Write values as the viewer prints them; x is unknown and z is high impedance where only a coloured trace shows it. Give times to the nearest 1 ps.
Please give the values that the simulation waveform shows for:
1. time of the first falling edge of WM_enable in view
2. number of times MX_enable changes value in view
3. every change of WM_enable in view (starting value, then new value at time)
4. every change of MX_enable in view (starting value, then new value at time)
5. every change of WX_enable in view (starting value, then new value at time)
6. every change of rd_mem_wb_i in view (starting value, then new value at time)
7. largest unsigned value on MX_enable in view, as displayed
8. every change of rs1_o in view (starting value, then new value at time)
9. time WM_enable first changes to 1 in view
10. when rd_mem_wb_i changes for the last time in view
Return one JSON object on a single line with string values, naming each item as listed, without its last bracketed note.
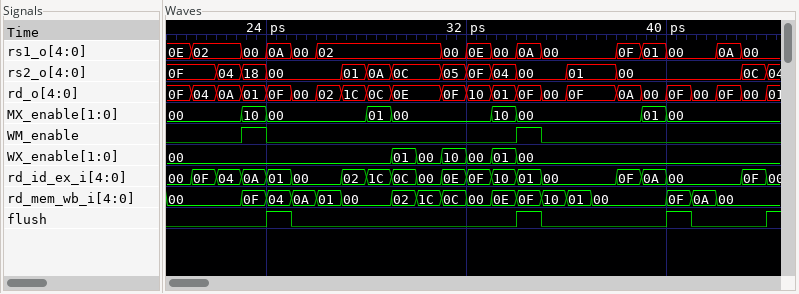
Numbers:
{"time of the first falling edge of WM_enable in view": "24 ps", "number of times MX_enable changes value in view": "8", "every change of WM_enable in view": "0, 1 at 23 ps, 0 at 24 ps, 1 at 34 ps, 0 at 35 ps", "every change of MX_enable in view": "00, 10 at 23 ps, 00 at 24 ps, 01 at 28 ps, 00 at 29 ps, 10 at 33 ps, 00 at 34 ps, 01 at 39 ps, 00 at 40 ps", "every change of WX_enable in view": "00, 01 at 29 ps, 00 at 30 ps, 10 at 31 ps, 00 at 32 ps, 01 at 33 ps, 00 at 34 ps", "every change of rd_mem_wb_i in view": "00, 0F at 23 ps, 04 at 24 ps, 0A at 25 ps, 01 at 26 ps, 00 at 27 ps, 02 at 29 ps, 1C at 30 ps, 0C at 31 ps, 00 at 32 ps, 0E at 33 ps, 0F at 34 ps, 10 at 35 ps, 01 at 36 ps, 00 at 37 ps, 0F at 40 ps, 0A at 41 ps, 00 at 42 ps", "largest unsigned value on MX_enable in view, as displayed": "10", "every change of rs1_o in view": "0E, 02 at 21 ps, 00 at 23 ps, 0A at 24 ps, 00 at 25 ps, 02 at 26 ps, 00 at 31 ps, 0E at 32 ps, 00 at 33 ps, 0A at 34 ps, 00 at 35 ps, 0F at 38 ps, 01 at 39 ps, 00 at 40 ps, 0A at 42 ps, 00 at 43 ps", "time WM_enable first changes to 1 in view": "23 ps", "when rd_mem_wb_i changes for the last time in view": "42 ps"}
